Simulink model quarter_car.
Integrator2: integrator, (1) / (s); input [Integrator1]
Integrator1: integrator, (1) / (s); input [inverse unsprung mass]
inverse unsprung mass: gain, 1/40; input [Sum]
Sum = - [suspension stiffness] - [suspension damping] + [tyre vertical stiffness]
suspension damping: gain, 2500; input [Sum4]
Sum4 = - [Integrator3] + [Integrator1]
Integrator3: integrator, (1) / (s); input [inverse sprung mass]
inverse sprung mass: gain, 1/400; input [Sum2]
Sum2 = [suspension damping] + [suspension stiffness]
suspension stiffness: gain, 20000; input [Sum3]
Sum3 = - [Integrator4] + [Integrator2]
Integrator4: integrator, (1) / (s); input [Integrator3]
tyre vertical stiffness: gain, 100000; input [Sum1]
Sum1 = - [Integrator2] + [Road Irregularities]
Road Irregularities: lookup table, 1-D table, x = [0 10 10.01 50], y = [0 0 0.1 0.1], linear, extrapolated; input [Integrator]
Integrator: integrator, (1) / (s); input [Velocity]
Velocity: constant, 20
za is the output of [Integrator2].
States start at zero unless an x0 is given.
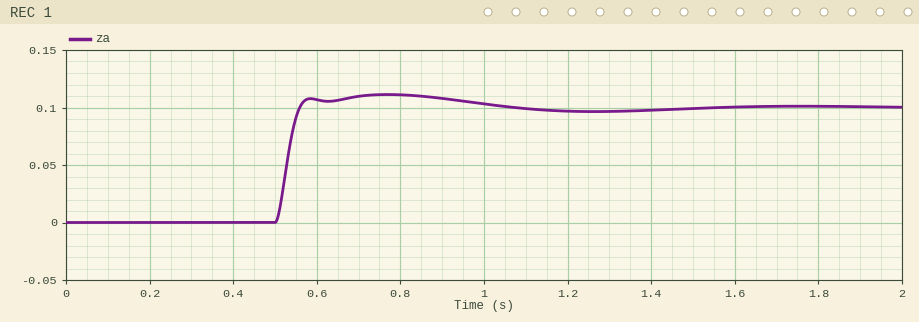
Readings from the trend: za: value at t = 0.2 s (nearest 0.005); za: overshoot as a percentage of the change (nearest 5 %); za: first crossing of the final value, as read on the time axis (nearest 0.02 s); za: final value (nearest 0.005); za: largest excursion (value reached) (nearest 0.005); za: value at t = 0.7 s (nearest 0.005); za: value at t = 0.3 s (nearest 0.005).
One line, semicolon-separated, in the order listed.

0.000; 10 %; 0.56 s; 0.100; 0.110; 0.110; 0.000
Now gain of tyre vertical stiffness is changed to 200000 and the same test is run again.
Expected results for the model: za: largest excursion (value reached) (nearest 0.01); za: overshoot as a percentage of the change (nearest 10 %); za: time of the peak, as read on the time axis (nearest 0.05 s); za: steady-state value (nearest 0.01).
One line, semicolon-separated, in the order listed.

0.12; 20 %; 0.55 s; 0.10
